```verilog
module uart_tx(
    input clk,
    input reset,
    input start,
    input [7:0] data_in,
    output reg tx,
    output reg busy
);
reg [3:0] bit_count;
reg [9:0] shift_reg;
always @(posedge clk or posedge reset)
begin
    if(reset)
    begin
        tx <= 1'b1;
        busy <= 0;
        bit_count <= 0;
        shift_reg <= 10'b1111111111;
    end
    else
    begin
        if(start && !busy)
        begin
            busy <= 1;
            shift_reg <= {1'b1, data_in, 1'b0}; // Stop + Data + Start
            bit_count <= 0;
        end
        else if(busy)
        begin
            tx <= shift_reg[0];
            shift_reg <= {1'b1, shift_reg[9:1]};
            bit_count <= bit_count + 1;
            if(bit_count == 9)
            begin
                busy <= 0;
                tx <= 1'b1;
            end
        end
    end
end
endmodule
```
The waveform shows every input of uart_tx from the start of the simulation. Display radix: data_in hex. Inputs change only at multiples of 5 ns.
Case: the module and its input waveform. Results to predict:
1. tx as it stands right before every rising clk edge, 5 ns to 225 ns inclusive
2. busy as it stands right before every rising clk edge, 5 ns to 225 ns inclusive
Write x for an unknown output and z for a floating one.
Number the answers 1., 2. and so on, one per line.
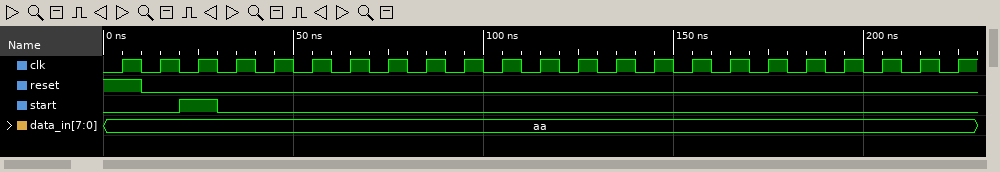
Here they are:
1. 1 1 1 1 0 0 1 0 1 0 1 0 1 1 1 1 1 1 1 1 1 1 1
2. 0 0 0 1 1 1 1 1 1 1 1 1 1 0 0 0 0 0 0 0 0 0 0
